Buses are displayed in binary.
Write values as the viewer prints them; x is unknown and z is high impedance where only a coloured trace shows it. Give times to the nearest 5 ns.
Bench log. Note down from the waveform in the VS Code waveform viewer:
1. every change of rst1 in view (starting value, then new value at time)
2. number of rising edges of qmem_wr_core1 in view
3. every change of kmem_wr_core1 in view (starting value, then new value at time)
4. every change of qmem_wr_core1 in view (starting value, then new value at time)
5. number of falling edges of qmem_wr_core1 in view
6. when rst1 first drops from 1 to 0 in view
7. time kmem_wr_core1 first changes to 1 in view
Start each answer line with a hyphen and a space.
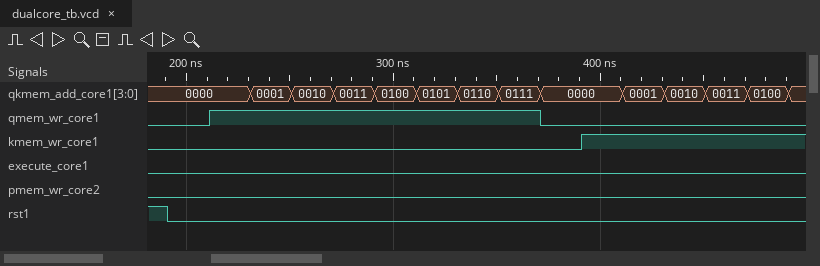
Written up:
- 1, 0 at 190 ns
- 1
- 0, 1 at 390 ns
- 0, 1 at 210 ns, 0 at 370 ns
- 1
- 190 ns
- 390 ns
